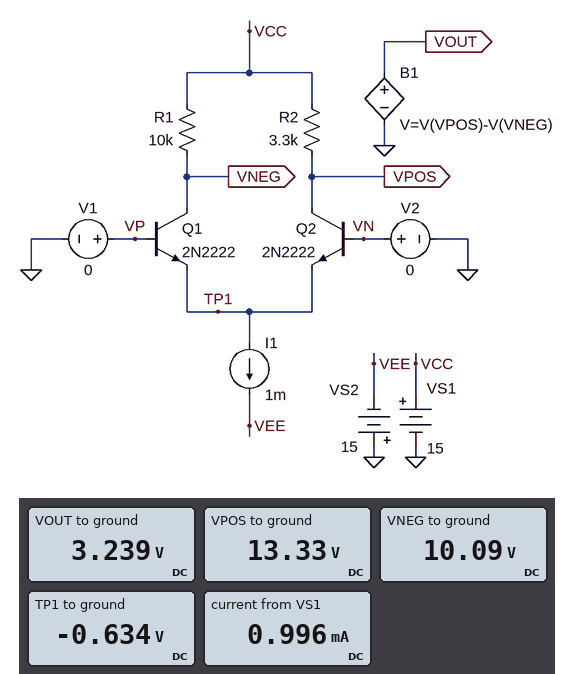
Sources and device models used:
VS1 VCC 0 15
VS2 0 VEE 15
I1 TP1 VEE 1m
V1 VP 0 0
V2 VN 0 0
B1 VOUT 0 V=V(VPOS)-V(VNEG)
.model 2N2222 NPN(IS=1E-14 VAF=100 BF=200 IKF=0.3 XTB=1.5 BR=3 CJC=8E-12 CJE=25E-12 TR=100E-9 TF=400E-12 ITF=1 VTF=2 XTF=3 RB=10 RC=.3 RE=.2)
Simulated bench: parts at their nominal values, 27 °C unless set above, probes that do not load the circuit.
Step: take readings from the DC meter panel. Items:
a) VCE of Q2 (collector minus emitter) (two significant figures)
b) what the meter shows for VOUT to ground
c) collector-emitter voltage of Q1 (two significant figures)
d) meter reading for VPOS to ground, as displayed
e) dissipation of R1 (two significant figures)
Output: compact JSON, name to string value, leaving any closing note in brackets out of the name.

{"VCE of Q2 (collector minus emitter)": "14 V", "what the meter shows for VOUT to ground": "3.239 V", "collector-emitter voltage of Q1": "11 V", "meter reading for VPOS to ground, as displayed": "13.33 V", "dissipation of R1": "2.4 mW"}
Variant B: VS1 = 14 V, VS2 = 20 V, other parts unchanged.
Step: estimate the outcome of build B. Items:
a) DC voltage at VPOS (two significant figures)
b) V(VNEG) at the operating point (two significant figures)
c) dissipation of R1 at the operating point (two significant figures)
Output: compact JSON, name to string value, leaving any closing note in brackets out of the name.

{"DC voltage at VPOS": "12 V", "V(VNEG) at the operating point": "9.1 V", "dissipation of R1 at the operating point": "2.4 mW"}
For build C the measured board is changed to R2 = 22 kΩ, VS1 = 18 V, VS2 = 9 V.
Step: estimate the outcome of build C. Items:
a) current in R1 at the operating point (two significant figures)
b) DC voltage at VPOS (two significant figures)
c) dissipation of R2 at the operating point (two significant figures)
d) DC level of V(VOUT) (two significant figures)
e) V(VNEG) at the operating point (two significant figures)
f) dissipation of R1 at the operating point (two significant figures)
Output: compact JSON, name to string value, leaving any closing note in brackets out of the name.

{"current in R1 at the operating point": "510 µA", "DC voltage at VPOS": "7.3 V", "dissipation of R2 at the operating point": "5.2 mW", "DC level of V(VOUT)": "-5.6 V", "V(VNEG) at the operating point": "13 V", "dissipation of R1 at the operating point": "2.6 mW"}
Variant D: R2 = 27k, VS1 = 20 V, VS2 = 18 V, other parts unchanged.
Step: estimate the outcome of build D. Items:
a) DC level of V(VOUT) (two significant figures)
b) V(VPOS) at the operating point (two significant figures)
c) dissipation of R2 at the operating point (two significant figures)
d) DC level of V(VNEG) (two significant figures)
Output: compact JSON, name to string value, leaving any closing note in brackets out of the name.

{"DC level of V(VOUT)": "-7.8 V", "V(VPOS) at the operating point": "7.0 V", "dissipation of R2 at the operating point": "6.2 mW", "DC level of V(VNEG)": "15 V"}
